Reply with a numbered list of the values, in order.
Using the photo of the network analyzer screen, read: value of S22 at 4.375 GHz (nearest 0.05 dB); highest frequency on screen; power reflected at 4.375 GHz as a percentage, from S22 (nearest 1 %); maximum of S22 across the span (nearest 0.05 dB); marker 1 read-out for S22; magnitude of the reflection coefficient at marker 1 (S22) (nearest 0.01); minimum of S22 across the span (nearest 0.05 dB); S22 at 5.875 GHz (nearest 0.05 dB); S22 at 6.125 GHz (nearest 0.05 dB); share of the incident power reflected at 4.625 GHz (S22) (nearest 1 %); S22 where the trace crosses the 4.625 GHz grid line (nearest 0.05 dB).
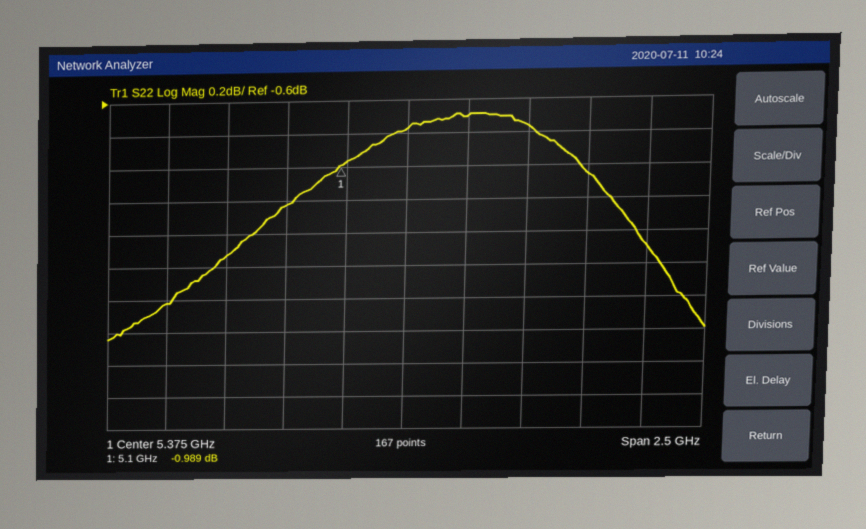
1. -1.80 dB
2. 6.625 GHz
3. 66 %
4. -0.70 dB
5. -0.989 dB
6. 0.89
7. -2.05 dB
8. -0.75 dB
9. -1.05 dB
10. 70 %
11. -1.55 dB
